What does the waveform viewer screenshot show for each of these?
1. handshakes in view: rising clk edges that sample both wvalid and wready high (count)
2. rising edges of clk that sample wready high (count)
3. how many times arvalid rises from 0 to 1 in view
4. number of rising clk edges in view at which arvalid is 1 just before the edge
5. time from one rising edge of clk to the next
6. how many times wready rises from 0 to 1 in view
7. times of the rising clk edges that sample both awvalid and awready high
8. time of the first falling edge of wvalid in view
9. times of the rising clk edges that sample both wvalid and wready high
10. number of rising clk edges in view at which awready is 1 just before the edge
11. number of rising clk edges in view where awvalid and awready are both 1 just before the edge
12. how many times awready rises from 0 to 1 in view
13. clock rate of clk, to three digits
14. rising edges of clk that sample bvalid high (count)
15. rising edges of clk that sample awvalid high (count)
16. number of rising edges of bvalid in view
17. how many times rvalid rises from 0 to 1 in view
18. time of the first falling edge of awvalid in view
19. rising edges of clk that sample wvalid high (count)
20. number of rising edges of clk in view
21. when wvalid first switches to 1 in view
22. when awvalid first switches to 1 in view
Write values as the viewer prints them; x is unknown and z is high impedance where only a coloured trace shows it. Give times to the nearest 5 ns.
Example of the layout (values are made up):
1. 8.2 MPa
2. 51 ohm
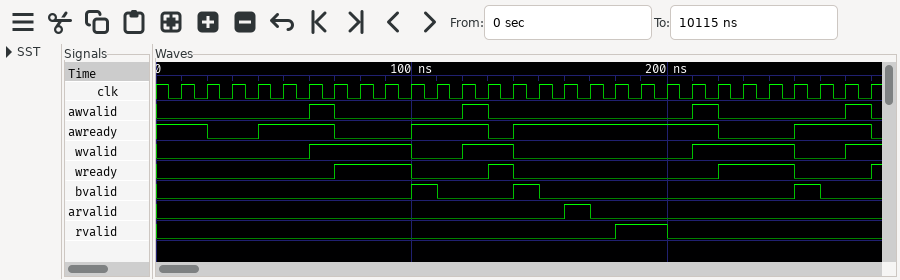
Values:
1. 7
2. 7
3. 1
4. 1
5. 10 ns
6. 4
7. 70 ns, 130 ns, 220 ns, 280 ns
8. 100 ns
9. 80 ns, 90 ns, 100 ns, 140 ns, 230 ns, 240 ns, 250 ns
10. 19
11. 4
12. 4
13. 100 MHz
14. 3
15. 4
16. 3
17. 1
18. 70 ns
19. 11
20. 28
21. 60 ns
22. 60 ns
